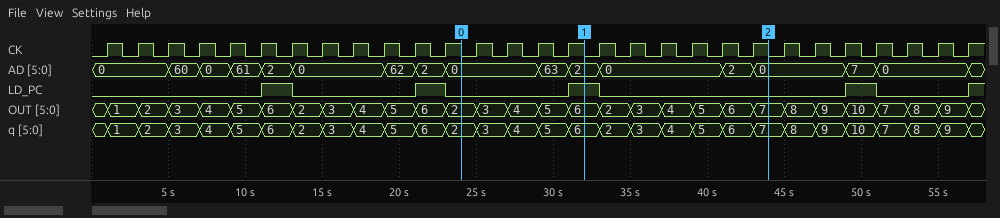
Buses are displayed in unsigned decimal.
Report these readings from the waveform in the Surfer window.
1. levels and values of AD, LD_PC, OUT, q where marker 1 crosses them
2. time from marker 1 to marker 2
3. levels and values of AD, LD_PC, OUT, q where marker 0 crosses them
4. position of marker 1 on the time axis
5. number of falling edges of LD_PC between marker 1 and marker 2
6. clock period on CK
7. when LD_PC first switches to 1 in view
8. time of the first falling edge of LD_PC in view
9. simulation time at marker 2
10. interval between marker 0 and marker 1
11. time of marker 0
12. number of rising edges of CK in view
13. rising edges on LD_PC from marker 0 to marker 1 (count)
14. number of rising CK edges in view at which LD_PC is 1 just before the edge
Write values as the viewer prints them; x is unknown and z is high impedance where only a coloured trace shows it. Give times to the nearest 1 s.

AD=2, LD_PC=1, OUT=6, q=6
12 s
AD=0, LD_PC=0, OUT=2, q=2
32 s
1
2 s
11 s
13 s
44 s
8 s
24 s
29
1
4
